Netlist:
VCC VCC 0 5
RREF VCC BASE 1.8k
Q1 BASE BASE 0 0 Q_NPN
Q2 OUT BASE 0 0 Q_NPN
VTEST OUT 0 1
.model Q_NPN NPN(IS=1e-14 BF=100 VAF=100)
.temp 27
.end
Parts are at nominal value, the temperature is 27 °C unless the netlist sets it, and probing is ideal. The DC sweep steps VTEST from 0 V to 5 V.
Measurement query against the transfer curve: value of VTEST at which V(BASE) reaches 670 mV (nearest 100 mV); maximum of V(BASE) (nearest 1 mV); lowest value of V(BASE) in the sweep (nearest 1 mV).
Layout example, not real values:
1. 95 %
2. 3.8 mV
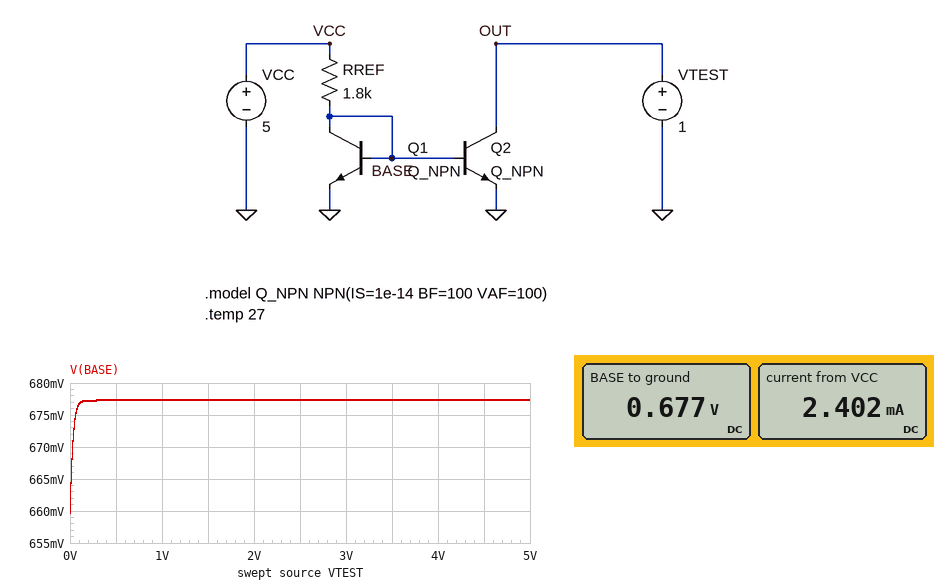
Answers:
1. 0 V
2. 677 mV
3. 660 mV
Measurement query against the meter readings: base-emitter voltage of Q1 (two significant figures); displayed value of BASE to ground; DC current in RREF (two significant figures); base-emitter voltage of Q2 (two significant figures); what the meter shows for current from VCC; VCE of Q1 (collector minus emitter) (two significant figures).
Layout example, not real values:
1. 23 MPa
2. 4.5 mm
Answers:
1. 680 mV
2. 0.677 V
3. 2.4 mA
4. 680 mV
5. 2.402 mA
6. 680 mV
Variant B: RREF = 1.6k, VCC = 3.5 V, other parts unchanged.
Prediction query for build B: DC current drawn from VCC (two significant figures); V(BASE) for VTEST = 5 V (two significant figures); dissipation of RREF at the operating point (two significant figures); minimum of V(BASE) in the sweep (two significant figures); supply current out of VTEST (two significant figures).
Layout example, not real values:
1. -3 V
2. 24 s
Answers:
1. 1.8 mA
2. 670 mV
3. 5.0 mW
4. 650 mV
5. 1.7 mA
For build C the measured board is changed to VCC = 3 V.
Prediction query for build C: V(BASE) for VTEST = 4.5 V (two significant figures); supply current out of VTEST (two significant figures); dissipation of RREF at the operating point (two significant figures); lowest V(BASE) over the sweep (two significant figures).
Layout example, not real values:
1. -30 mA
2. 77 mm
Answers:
1. 660 mV
2. 1.3 mA
3. 3.0 mW
4. 640 mV
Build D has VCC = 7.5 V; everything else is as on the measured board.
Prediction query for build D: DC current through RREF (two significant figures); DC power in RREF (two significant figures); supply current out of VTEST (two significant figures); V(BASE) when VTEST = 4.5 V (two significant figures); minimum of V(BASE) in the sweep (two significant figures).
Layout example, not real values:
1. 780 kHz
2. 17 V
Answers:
1. 3.8 mA
2. 26 mW
3. 3.7 mA
4. 690 mV
5. 670 mV
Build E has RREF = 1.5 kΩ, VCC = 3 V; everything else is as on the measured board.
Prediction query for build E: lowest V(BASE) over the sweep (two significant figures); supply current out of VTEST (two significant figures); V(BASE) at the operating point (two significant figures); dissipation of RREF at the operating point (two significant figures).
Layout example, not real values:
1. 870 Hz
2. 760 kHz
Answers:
1. 650 mV
2. 1.5 mA
3. 670 mV
4. 3.6 mW
